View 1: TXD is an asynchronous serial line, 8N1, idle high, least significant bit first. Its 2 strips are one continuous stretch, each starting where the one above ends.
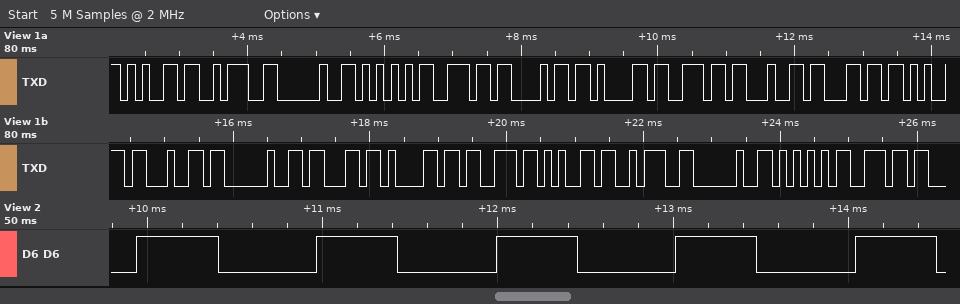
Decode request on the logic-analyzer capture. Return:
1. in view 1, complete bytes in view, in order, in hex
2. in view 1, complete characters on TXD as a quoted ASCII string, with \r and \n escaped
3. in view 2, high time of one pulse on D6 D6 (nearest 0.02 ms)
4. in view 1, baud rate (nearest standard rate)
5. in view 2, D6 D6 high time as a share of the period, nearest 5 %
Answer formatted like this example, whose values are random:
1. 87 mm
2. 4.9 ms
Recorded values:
1. 65 3A 20 55 6E 68 61 6E 64 6C 65 64 20 63 61 73 65 3A 20 55 6E
2. "e: Unhandled case: Un"
3. 0.46 ms
4. 9600 baud
5. 45 %
